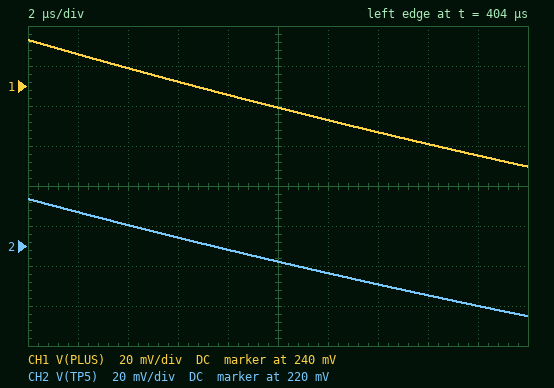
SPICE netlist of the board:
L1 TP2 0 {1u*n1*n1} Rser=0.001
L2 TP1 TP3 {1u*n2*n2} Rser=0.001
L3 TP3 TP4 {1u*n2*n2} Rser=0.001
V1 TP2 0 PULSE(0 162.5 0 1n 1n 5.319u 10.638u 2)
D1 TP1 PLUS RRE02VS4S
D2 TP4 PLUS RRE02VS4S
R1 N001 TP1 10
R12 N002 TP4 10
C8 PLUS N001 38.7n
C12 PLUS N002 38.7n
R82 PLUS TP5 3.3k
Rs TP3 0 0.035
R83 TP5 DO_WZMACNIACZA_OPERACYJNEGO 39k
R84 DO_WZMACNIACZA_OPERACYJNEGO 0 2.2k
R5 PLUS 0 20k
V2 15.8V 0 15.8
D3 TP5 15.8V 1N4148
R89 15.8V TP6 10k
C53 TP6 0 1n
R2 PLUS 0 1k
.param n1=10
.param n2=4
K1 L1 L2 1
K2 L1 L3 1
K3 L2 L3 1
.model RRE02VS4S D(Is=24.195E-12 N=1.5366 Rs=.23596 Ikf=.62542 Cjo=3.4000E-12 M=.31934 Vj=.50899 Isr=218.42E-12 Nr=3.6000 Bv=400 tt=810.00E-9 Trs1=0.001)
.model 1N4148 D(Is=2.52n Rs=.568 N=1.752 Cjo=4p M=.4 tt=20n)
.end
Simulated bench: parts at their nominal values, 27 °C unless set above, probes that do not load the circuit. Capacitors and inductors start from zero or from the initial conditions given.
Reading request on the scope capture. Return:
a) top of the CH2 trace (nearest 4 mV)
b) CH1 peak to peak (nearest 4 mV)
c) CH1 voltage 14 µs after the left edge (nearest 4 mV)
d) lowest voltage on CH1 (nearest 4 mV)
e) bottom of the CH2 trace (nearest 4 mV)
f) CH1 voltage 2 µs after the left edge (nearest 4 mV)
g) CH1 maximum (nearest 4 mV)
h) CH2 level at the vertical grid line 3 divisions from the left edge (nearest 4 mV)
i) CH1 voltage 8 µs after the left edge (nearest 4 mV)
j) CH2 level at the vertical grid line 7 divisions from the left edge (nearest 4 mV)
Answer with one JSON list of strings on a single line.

["244 mV", "64 mV", "216 mV", "200 mV", "184 mV", "256 mV", "264 mV", "224 mV", "236 mV", "200 mV"]
